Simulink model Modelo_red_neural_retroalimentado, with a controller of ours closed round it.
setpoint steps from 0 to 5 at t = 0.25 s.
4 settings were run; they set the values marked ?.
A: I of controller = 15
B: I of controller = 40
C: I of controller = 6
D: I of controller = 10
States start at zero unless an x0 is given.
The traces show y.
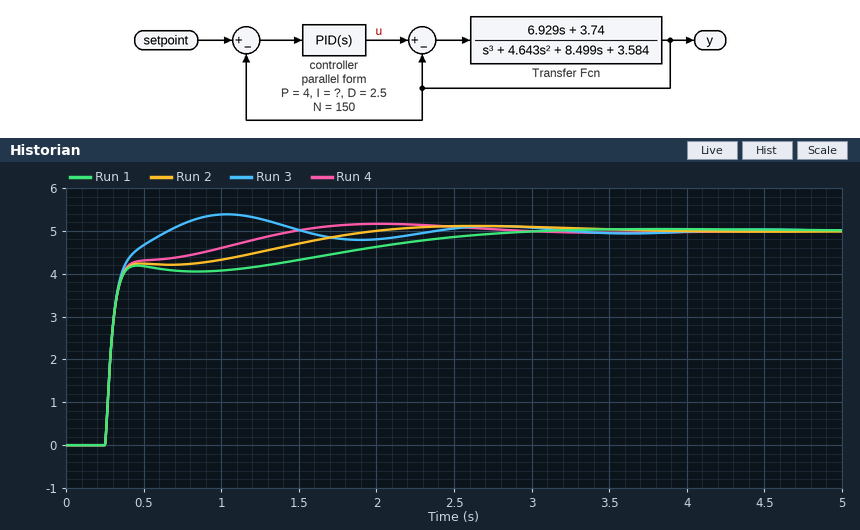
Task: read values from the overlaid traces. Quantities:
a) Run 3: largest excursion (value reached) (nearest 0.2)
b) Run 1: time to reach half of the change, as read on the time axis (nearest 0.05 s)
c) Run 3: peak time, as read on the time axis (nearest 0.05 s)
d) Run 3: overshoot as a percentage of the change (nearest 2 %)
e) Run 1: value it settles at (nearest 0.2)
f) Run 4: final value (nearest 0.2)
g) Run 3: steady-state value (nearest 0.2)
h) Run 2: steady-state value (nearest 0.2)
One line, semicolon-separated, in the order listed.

5.4; 0.30 s; 1.05 s; 8 %; 5.0; 5.0; 5.0; 5.0
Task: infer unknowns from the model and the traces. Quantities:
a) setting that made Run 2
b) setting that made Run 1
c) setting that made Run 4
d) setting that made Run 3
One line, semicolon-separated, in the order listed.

D; C; A; B
